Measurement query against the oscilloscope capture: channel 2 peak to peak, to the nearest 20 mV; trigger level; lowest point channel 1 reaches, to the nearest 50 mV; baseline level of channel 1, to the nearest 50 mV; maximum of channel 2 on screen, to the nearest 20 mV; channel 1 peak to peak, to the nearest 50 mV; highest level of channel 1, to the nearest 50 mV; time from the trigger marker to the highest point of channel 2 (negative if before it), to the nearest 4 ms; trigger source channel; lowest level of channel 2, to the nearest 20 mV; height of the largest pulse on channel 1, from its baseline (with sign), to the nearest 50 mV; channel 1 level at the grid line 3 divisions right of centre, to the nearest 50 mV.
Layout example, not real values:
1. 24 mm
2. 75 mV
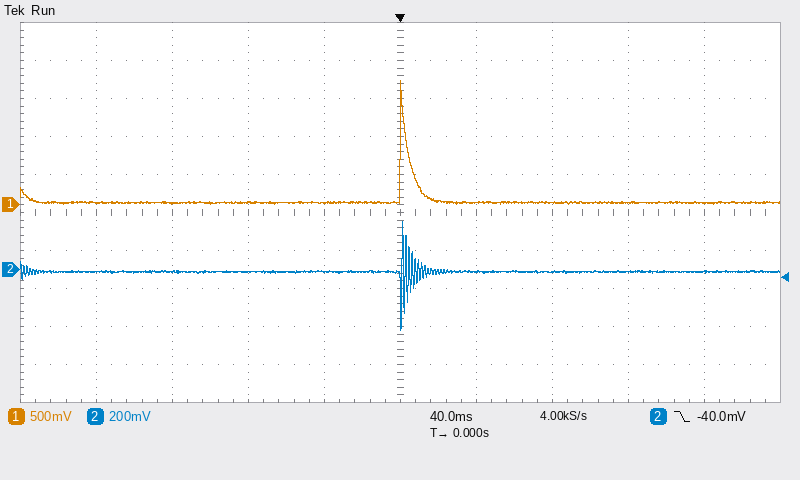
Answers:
1. 580 mV
2. -40.0 mV
3. 0 mV
4. 50 mV
5. 260 mV
6. 1.65 V
7. 1.65 V
8. 0 ms
9. channel 2
10. -320 mV
11. +1.60 V
12. 50 mV
